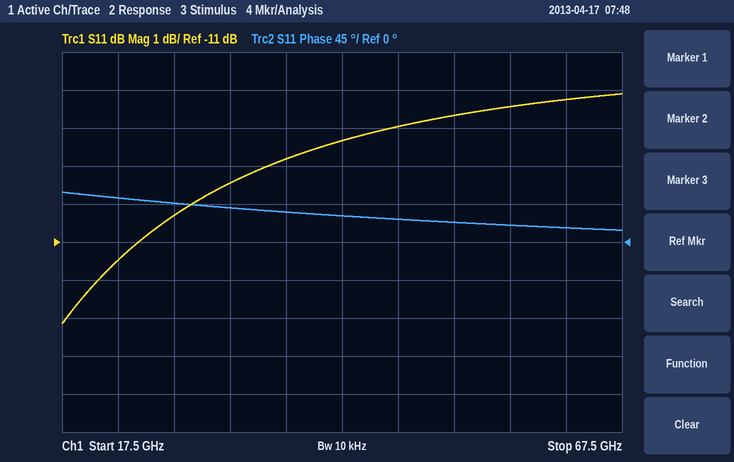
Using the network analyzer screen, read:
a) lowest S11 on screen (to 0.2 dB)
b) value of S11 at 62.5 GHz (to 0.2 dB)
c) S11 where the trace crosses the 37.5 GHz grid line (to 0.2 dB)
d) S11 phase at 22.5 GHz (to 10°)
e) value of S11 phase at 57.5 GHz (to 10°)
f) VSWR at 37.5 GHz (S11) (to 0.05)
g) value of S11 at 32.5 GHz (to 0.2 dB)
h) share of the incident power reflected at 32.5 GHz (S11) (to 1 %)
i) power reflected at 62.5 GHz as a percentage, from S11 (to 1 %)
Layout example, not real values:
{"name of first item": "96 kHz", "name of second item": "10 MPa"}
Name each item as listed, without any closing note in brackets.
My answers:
{"lowest S11 on screen": "-13.2 dB", "value of S11 at 62.5 GHz": "-7.2 dB", "S11 where the trace crosses the 37.5 GHz grid line": "-8.8 dB", "S11 phase at 22.5 GHz": "50°", "value of S11 phase at 57.5 GHz": "20°", "VSWR at 37.5 GHz (S11)": "2.15", "value of S11 at 32.5 GHz": "-9.4 dB", "share of the incident power reflected at 32.5 GHz (S11)": "11 %", "power reflected at 62.5 GHz as a percentage, from S11": "19 %"}
